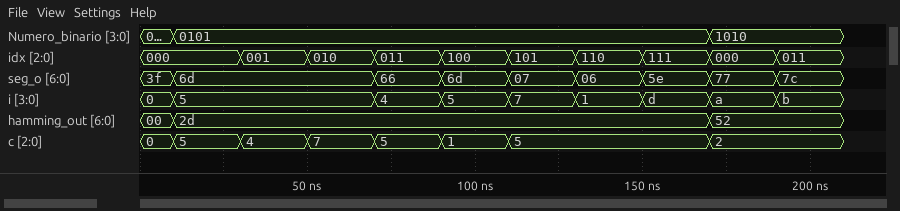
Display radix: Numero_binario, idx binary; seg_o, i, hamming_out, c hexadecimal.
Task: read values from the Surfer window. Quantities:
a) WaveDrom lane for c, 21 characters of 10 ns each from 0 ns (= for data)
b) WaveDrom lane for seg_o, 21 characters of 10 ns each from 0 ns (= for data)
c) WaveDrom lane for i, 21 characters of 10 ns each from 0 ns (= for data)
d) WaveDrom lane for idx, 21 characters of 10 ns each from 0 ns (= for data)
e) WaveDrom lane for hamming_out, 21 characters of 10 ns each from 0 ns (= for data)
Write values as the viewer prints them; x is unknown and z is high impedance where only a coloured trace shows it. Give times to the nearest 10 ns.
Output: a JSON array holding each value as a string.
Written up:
["{name: 'c', wave: '==.=.=.=.=.=.....=...', data: '0 5 4 7 5 1 5 2'}", "{name: 'seg_o', wave: '==.....=.=.=.=.=.=.=.', data: '3f 6d 66 6d 07 06 5e 77 7c'}", "{name: 'i', wave: '==.....=.=.=.=.=.=.=.', data: '0 5 4 5 7 1 d a b'}", "{name: 'idx', wave: '=..=.=.=.=.=.=.=.=.=.', data: '000 001 010 011 100 101 110 111 000 011'}", "{name: 'hamming_out', wave: '==...............=...', data: '00 2d 52'}"]
